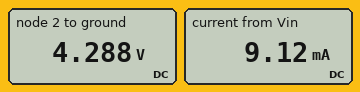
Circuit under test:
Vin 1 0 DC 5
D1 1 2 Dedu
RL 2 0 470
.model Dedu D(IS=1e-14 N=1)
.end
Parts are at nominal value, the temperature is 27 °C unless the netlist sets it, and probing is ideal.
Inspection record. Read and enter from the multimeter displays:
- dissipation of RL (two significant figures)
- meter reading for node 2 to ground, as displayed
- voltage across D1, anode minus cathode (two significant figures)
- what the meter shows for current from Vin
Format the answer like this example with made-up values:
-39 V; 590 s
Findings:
39 mW; 4.288 V; 710 mV; 9.12 mA
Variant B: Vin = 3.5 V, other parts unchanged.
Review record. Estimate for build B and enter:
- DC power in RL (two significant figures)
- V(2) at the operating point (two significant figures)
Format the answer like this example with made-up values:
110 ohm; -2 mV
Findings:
17 mW; 2.8 V
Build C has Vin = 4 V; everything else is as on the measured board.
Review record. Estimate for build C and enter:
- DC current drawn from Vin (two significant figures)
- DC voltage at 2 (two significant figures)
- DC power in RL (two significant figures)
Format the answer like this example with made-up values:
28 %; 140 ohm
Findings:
7.0 mA; 3.3 V; 23 mW
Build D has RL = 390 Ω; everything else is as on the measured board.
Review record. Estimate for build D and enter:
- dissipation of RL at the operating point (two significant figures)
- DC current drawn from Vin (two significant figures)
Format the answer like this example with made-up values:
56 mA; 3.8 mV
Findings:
47 mW; 11 mA
